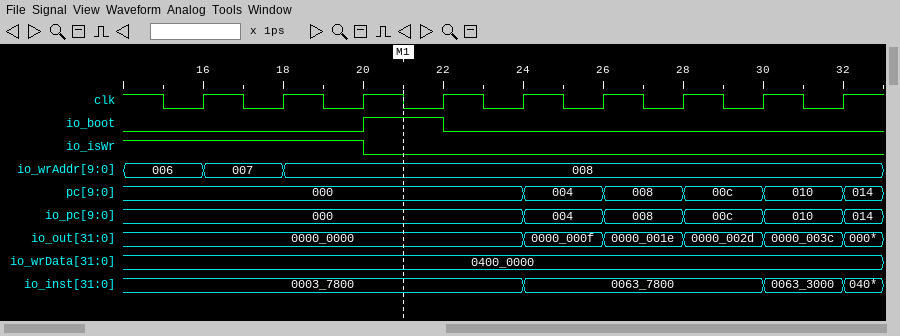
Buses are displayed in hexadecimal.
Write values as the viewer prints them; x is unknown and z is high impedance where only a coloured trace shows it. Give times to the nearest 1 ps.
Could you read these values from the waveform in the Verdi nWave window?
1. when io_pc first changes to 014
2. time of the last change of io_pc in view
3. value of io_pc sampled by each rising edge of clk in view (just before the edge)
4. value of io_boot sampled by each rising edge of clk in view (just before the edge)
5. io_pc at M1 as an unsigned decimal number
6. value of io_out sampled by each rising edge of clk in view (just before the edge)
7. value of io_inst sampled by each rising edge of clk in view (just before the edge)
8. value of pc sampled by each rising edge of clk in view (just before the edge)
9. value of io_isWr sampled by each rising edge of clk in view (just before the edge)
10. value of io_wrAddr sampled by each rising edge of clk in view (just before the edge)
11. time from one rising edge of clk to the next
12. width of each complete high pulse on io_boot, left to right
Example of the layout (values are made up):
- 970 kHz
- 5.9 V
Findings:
- 32 ps
- 32 ps
- 000, 000, 000, 000, 000, 004, 008, 00c, 010
- 0 0 0 1 0 0 0 0 0
- 0
- 0000_0000, 0000_0000, 0000_0000, 0000_0000, 0000_0000, 0000_000f, 0000_001e, 0000_002d, 0000_003c
- 0003_7800, 0003_7800, 0003_7800, 0003_7800, 0003_7800, 0063_7800, 0063_7800, 0063_7800, 0063_3000
- 000, 000, 000, 000, 000, 004, 008, 00c, 010
- 1 1 1 0 0 0 0 0 0
- 006, 007, 008, 008, 008, 008, 008, 008, 008
- 2 ps
- 2 ps
